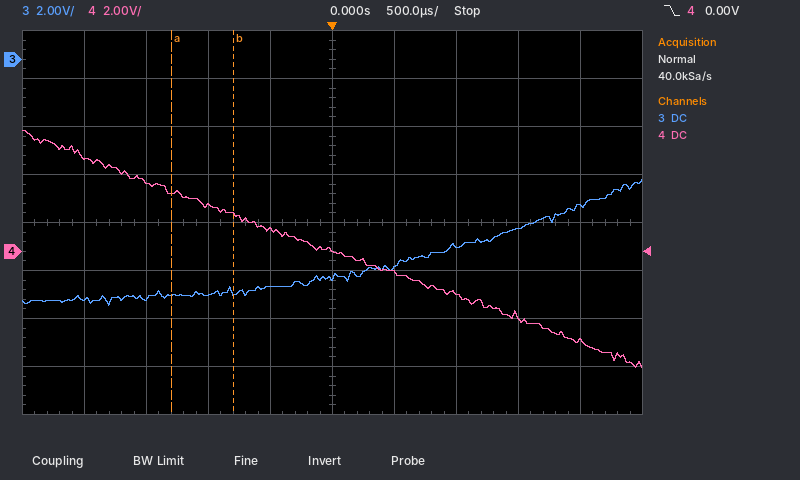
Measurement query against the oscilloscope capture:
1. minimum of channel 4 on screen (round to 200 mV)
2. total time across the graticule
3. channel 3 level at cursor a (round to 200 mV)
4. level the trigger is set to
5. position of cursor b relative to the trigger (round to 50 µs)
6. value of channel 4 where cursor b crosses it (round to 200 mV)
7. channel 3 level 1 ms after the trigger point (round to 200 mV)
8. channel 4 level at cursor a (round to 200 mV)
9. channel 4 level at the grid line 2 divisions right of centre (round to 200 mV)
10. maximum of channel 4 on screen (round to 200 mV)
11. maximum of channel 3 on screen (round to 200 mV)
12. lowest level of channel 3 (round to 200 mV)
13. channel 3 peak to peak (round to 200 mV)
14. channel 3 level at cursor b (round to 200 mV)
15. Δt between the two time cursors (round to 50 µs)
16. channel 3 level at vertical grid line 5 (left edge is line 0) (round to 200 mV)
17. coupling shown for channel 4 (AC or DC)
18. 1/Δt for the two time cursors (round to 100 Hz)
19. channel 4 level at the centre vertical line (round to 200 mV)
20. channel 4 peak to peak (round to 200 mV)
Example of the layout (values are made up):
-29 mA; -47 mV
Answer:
-4.8 V; 5 ms; -9.8 V; 0.00 V; -800 µs; 1.6 V; -7.8 V; 2.4 V; -1.8 V; 5.0 V; -5.0 V; -10.2 V; 5.2 V; -9.6 V; 500 µs; -9.0 V; DC; 2.0 kHz; 0.0 V; 9.8 V
